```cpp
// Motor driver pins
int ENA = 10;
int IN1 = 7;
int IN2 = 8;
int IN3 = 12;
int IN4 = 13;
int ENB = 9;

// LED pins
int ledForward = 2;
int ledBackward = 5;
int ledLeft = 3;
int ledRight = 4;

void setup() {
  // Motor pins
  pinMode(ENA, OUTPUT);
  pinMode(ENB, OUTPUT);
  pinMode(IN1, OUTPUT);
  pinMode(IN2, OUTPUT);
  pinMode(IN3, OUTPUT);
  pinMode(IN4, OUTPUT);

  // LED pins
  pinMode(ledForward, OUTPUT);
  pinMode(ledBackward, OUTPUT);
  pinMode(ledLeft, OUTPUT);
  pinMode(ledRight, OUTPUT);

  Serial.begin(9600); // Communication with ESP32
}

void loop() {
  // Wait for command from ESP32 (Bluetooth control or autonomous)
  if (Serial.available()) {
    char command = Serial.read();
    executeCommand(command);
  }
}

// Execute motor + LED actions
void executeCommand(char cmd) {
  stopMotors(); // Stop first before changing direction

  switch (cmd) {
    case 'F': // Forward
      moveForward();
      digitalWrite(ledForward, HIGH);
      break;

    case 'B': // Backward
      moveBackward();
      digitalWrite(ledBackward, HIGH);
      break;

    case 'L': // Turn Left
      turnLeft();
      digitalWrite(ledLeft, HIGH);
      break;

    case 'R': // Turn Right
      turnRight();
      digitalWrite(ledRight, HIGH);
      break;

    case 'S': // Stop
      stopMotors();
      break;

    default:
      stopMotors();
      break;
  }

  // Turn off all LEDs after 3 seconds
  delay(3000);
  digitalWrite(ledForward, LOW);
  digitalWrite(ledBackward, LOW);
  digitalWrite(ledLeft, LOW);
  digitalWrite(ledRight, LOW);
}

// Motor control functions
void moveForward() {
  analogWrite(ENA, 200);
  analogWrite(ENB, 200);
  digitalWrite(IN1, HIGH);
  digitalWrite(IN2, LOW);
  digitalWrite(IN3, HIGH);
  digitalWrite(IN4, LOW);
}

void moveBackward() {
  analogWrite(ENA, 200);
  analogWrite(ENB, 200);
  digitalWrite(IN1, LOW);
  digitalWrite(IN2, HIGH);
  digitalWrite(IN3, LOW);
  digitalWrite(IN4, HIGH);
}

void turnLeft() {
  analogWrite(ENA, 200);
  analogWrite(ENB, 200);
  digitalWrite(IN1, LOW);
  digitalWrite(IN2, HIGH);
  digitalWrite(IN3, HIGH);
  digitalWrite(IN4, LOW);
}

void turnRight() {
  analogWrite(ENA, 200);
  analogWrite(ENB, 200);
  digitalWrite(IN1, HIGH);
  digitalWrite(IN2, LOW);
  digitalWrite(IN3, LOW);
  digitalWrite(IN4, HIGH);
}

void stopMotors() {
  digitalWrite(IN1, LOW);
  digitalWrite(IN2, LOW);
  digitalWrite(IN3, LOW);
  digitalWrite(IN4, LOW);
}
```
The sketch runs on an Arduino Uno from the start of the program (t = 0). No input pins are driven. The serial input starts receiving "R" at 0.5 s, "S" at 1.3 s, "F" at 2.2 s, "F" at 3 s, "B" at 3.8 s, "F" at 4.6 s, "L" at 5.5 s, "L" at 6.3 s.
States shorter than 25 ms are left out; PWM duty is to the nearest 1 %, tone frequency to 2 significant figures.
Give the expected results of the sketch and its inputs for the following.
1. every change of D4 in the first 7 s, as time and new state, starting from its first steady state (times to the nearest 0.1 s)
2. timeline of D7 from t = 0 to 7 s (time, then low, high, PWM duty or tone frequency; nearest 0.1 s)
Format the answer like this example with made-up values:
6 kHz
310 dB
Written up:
0 s low; 0.5 s high; 3.5 s low
0 s low; 0.5 s high; 3.5 s low; 6.5 s high
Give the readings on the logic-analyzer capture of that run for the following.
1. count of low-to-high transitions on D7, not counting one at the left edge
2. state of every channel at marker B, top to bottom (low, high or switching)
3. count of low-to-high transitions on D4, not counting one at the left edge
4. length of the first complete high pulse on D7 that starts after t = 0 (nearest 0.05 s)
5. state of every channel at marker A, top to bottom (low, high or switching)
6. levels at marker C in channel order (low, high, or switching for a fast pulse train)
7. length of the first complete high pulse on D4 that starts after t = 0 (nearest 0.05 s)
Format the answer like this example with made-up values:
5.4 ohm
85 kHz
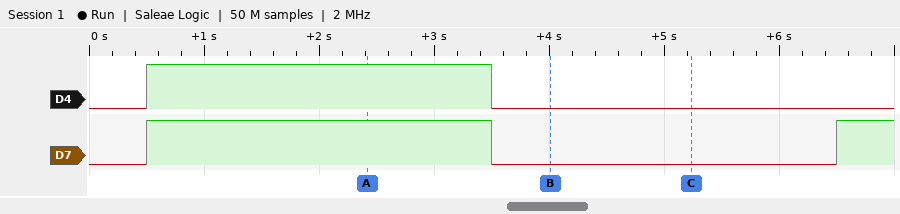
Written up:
2
D4 low, D7 low
1
3.00 s
D4 high, D7 high
D4 low, D7 low
3.00 s
